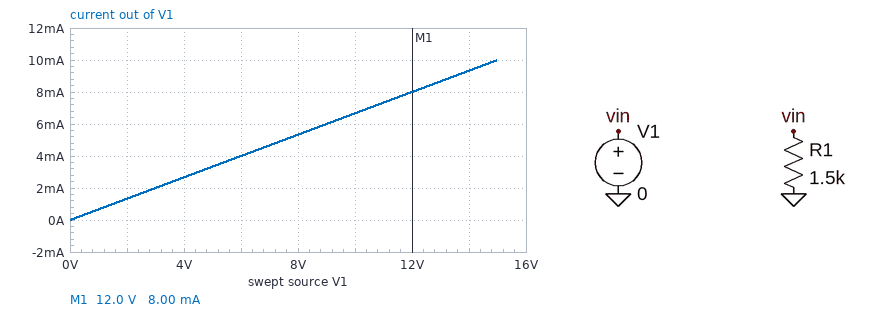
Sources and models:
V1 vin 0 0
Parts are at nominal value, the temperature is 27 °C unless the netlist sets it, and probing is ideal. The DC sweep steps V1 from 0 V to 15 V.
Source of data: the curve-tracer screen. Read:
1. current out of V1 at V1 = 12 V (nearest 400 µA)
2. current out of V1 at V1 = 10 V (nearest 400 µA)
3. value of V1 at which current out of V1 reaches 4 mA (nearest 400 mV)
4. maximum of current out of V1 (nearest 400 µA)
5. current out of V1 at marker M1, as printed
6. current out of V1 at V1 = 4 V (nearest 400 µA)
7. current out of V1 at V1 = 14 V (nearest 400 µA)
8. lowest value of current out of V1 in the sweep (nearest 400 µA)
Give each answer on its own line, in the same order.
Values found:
8.0 mA
6.8 mA
6.0 V
10.0 mA
8.00 mA
2.8 mA
9.2 mA
0 A
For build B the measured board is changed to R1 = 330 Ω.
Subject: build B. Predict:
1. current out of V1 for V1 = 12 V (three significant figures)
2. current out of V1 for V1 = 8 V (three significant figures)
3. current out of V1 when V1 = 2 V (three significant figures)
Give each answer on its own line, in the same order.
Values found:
36.4 mA
24.2 mA
6.06 mA
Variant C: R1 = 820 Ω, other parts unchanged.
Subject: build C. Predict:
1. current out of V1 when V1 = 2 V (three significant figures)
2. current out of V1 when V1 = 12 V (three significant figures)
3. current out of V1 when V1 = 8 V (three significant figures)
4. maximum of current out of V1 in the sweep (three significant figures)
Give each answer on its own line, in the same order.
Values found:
2.44 mA
14.6 mA
9.76 mA
18.3 mA
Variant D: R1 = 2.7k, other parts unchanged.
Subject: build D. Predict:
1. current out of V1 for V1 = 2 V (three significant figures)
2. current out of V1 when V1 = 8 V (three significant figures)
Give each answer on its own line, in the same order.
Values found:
741 µA
2.96 mA
